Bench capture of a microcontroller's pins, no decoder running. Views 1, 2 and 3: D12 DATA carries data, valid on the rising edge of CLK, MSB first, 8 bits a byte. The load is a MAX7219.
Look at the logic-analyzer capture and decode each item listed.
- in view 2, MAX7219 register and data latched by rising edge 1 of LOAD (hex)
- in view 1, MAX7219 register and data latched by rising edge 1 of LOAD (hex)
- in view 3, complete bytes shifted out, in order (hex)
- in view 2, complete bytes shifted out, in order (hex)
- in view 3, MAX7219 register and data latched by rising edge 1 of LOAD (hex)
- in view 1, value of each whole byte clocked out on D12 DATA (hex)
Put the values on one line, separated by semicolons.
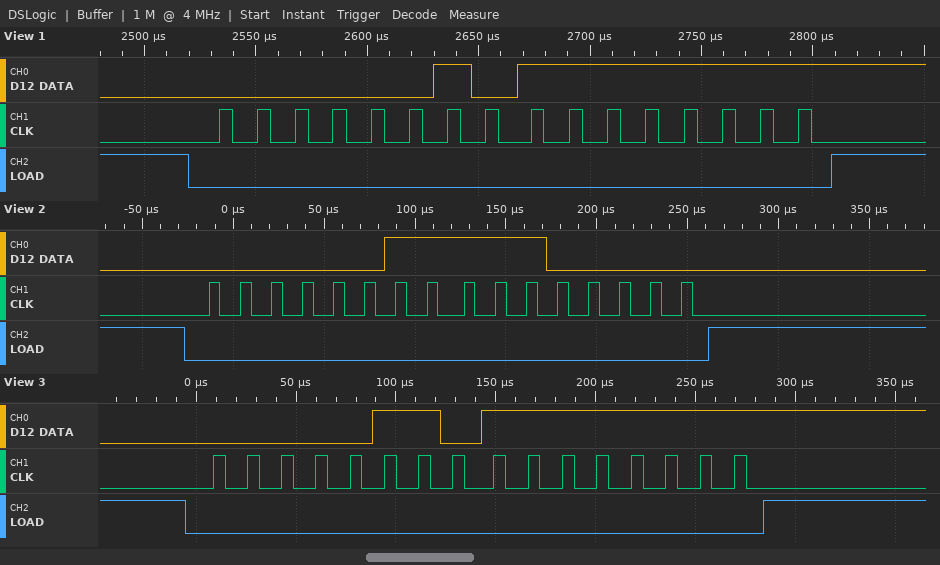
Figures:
register 0x3, data 0xE0; register 0x2, data 0xFF; 06 FF; 0x03 0xE0; register 0x6, data 0xFF; 02 FF
